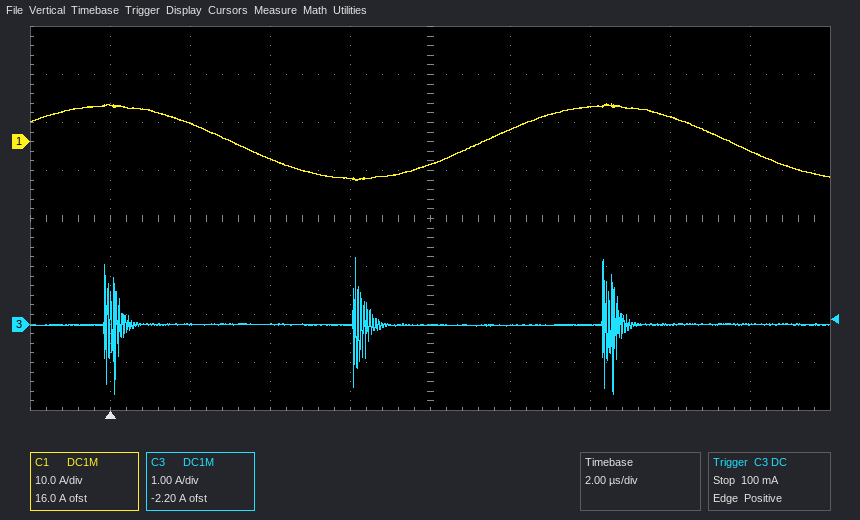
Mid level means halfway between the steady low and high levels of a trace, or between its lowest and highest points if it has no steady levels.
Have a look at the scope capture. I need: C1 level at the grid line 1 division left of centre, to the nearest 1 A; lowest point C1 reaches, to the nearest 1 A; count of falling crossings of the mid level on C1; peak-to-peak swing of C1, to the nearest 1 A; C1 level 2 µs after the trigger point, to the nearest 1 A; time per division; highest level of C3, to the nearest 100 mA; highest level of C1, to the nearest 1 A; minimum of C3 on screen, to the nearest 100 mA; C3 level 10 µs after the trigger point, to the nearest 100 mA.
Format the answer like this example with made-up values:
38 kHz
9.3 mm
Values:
-8 A
-8 A
2
16 A
4 A
2 µs
1.4 A
8 A
-1.5 A
0.0 A
